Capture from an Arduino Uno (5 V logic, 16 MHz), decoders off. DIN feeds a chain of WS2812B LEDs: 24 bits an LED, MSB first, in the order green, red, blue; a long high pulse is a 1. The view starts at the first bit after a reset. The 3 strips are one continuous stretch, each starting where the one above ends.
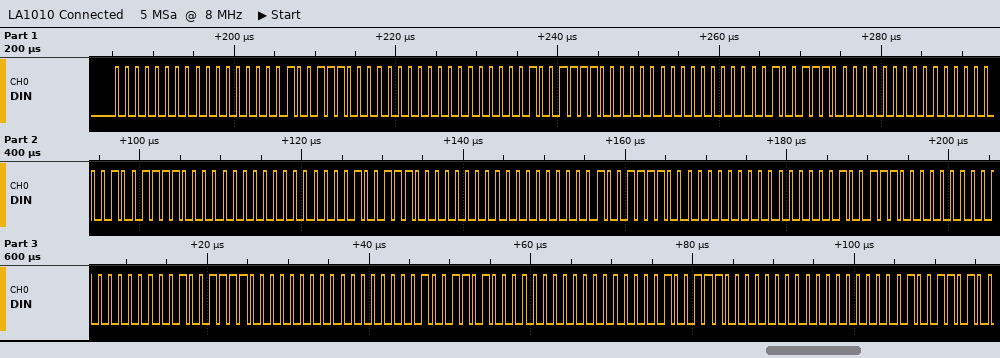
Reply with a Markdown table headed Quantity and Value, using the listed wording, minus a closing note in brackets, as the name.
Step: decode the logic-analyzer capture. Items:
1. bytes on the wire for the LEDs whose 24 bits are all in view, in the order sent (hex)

| Quantity | Value |
|---|---|
| bytes on the wire for the LEDs whose 24 bits are all in view, in the order sent | 00 00 4E 00 00 4F 00 00 4E 00 00 4F 00 00 4E 00 00 4F 00 00 4E 00 00 4F 00 00 4D 00 00 4E 00 00 4D |
